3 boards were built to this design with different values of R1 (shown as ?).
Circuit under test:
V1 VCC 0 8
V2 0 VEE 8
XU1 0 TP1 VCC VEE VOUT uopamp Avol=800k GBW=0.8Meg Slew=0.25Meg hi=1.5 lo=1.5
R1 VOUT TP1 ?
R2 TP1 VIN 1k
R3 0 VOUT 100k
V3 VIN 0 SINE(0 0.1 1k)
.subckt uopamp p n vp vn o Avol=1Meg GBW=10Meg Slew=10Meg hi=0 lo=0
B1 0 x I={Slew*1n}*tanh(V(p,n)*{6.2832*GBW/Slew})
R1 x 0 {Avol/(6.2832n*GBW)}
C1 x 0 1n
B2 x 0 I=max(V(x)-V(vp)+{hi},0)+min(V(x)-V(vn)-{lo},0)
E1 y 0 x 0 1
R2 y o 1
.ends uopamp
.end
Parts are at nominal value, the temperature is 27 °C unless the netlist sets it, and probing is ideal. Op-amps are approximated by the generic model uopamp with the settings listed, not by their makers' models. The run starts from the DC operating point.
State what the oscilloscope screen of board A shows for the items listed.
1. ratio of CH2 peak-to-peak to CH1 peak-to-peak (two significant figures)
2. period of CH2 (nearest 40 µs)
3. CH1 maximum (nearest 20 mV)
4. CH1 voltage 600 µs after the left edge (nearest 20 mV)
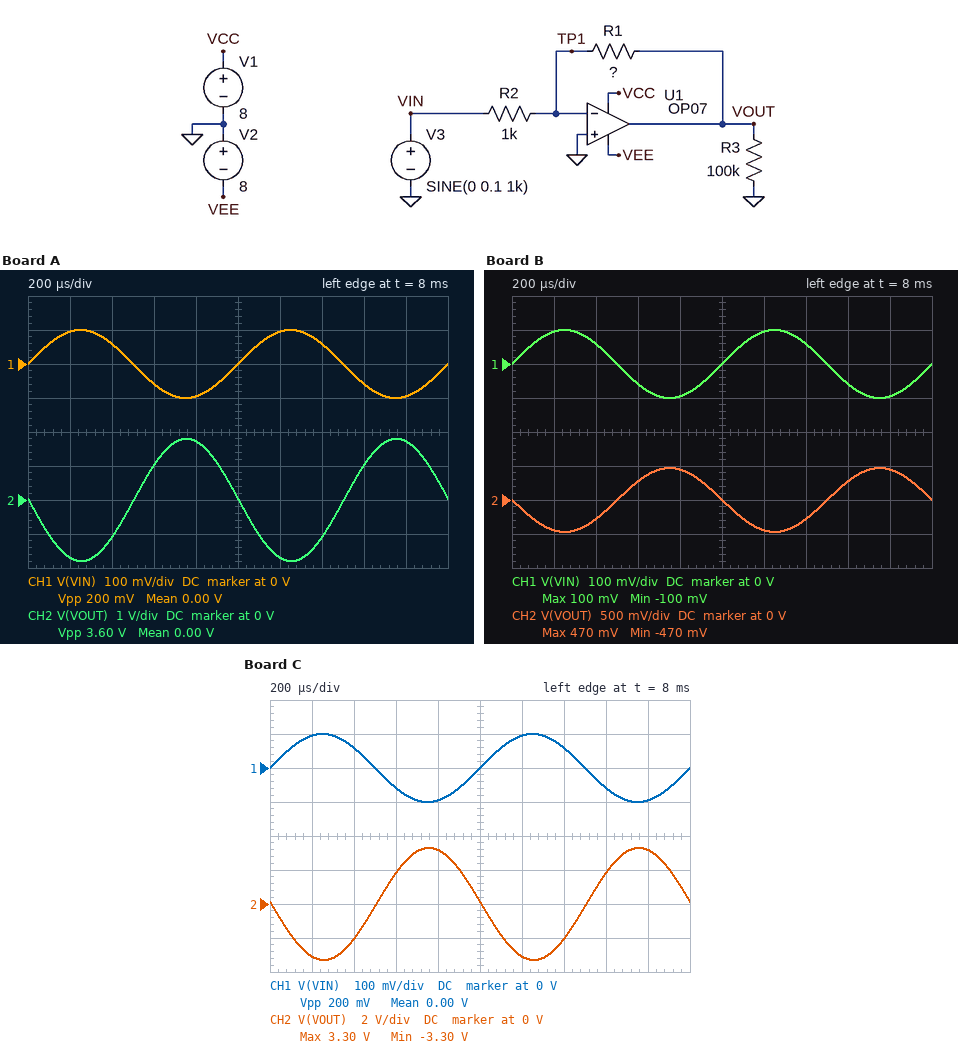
18
1.00 ms
100 mV
-60 mV
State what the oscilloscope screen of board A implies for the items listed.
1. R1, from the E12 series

18 kΩ
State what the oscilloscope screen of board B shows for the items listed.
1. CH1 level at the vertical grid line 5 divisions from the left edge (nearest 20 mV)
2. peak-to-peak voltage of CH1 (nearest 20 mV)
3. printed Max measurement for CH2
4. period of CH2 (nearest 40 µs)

0 V
200 mV
470 mV
1.00 ms
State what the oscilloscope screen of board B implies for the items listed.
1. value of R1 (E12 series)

4.7 kΩ
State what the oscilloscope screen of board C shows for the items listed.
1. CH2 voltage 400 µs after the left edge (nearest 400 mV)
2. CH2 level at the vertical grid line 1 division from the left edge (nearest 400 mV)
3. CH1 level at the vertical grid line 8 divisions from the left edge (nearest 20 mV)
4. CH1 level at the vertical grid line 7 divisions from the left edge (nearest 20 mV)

-2.0 V
-3.2 V
-60 mV
60 mV
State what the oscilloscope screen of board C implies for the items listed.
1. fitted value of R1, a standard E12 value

33 kΩ
